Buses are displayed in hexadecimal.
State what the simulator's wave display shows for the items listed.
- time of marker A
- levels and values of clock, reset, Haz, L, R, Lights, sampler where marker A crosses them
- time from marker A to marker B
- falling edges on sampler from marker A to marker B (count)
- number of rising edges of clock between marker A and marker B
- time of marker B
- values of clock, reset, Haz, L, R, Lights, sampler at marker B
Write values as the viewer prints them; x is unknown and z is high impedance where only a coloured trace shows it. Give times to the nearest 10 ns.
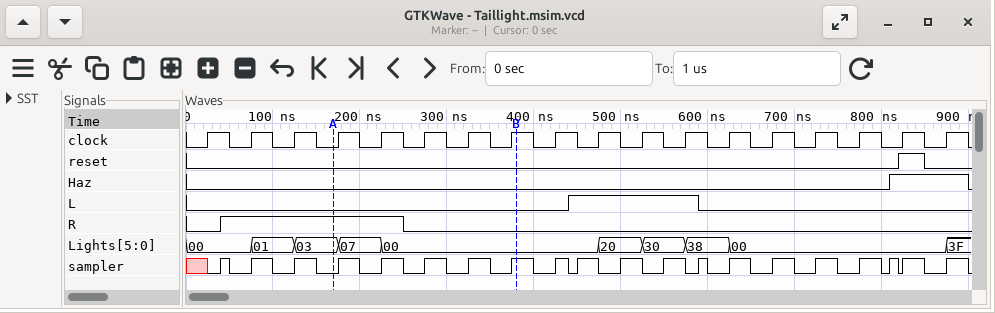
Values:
170 ns
clock=0, reset=0, Haz=0, L=0, R=1, Lights=03, sampler=0
210 ns
4
5
380 ns
clock=1, reset=0, Haz=0, L=0, R=0, Lights=00, sampler=1
